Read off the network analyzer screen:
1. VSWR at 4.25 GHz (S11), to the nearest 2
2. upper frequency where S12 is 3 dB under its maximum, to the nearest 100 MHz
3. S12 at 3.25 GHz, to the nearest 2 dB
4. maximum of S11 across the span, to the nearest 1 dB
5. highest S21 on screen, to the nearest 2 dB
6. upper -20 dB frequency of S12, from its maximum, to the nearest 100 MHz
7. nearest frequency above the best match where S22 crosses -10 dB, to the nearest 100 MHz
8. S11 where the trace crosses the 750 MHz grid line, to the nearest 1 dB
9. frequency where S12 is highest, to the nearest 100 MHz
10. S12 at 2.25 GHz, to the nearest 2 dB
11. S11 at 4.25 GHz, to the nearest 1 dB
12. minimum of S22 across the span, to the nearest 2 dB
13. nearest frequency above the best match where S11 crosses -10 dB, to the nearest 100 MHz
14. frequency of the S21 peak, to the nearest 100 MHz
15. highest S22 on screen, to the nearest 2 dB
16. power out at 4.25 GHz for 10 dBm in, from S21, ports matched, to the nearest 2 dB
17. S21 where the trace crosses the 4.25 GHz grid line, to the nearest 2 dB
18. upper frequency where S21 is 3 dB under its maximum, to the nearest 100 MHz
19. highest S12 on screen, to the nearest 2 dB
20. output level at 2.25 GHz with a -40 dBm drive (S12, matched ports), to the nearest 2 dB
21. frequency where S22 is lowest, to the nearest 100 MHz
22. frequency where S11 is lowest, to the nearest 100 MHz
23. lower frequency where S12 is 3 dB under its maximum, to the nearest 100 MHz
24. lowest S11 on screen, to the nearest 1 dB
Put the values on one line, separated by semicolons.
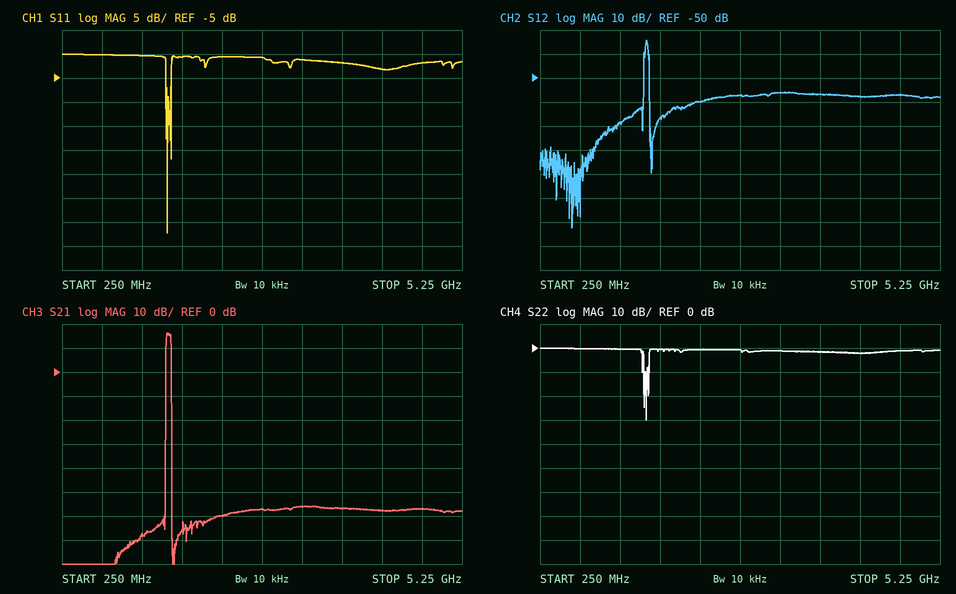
6; 1.6 GHz; -56 dB; 0 dB; 16 dB; 1.6 GHz; 1.6 GHz; 0 dB; 1.6 GHz; -60 dB; -3 dB; -30 dB; 1.6 GHz; 1.6 GHz; 0 dB; -48 dBm; -58 dB; 1.6 GHz; -34 dB; -100 dBm; 1.6 GHz; 1.6 GHz; 1.6 GHz; -37 dB
